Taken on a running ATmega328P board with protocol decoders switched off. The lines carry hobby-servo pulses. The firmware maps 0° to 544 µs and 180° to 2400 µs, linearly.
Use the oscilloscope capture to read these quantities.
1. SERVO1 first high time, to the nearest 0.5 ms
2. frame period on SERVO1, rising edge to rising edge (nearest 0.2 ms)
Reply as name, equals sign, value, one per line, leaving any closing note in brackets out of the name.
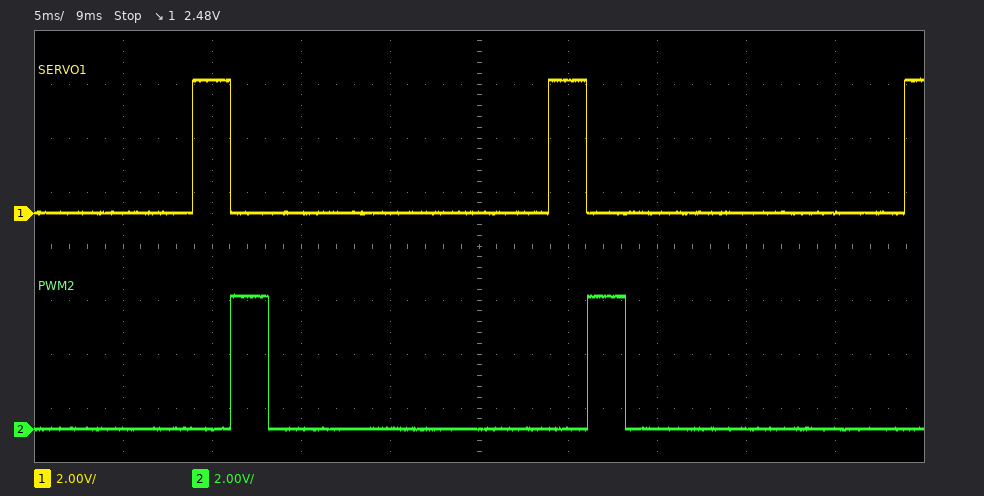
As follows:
SERVO1 first high time, to the nearest 0.5 ms = 2.0 ms
frame period on SERVO1, rising edge to rising edge = 20.0 ms
